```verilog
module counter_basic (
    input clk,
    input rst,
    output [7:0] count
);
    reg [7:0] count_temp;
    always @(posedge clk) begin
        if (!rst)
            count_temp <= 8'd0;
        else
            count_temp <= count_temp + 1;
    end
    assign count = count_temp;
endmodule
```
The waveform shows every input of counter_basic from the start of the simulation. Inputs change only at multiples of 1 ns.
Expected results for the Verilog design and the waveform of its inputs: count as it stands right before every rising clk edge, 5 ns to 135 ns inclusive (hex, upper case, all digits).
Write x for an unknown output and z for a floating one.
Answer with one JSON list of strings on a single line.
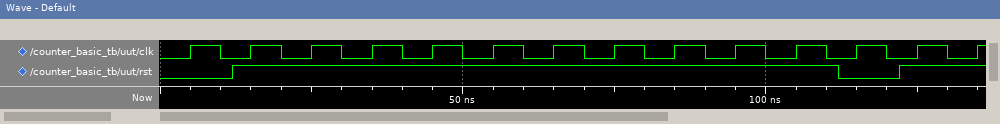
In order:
["x, 00, 01, 02, 03, 04, 05, 06, 07, 08, 09, 0A, 00, 01"]
